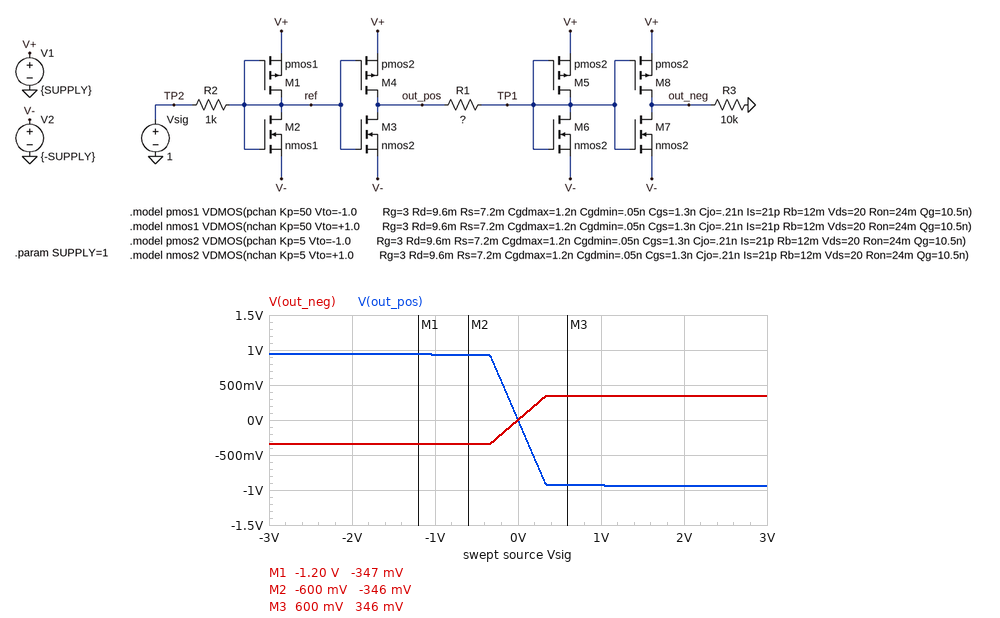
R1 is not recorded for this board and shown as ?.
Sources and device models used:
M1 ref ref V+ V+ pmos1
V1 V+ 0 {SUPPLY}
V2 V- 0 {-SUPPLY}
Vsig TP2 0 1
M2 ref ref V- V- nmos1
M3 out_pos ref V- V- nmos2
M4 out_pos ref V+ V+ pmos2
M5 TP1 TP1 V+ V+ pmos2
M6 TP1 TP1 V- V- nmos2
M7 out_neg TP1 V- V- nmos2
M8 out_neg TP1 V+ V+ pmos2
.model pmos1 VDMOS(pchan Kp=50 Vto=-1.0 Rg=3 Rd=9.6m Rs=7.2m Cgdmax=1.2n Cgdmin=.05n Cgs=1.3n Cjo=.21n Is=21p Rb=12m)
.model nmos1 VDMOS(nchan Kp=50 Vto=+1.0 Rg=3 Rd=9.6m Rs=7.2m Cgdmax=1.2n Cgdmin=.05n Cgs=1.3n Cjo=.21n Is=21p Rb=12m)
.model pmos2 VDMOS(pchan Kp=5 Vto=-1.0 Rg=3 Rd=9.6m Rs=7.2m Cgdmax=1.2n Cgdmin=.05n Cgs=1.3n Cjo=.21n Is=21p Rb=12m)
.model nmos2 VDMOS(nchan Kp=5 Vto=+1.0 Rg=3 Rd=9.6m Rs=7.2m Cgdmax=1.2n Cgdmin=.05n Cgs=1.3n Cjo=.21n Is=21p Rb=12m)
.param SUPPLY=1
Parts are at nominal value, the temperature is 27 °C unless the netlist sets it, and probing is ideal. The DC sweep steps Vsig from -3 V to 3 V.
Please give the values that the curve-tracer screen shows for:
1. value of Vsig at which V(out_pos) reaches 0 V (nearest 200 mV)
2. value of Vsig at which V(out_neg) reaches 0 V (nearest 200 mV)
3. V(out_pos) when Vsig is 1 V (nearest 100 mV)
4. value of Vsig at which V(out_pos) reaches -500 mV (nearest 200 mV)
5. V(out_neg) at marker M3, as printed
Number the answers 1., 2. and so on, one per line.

1. 0 V
2. 0 V
3. -900 mV
4. 200 mV
5. 346 mV
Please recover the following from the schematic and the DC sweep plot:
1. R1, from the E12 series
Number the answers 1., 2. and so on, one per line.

1. 27 kΩ
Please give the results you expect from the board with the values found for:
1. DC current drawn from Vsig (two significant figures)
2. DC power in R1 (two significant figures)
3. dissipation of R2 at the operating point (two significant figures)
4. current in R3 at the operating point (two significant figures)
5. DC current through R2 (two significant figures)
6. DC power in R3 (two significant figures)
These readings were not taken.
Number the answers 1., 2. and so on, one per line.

1. 1.0 mA
2. 32 µW
3. 1.0 mW
4. 35 µA
5. 1.0 mA
6. 12 µW
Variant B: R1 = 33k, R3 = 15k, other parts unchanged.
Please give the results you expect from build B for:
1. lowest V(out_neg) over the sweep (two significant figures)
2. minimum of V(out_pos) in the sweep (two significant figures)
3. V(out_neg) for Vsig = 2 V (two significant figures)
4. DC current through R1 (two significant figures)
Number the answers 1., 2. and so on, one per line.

1. -430 mV
2. -940 mV
3. 430 mV
4. 28 µA
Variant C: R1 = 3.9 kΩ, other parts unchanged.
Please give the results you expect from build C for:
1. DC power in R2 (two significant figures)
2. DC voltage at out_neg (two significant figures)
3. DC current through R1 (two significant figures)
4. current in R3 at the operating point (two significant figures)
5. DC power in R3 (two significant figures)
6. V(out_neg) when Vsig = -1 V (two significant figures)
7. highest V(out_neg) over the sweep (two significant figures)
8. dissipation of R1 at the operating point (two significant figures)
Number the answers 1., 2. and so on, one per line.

1. 1.0 mW
2. 930 mV
3. 100 µA
4. 93 µA
5. 87 µW
6. -930 mV
7. 940 mV
8. 41 µW
